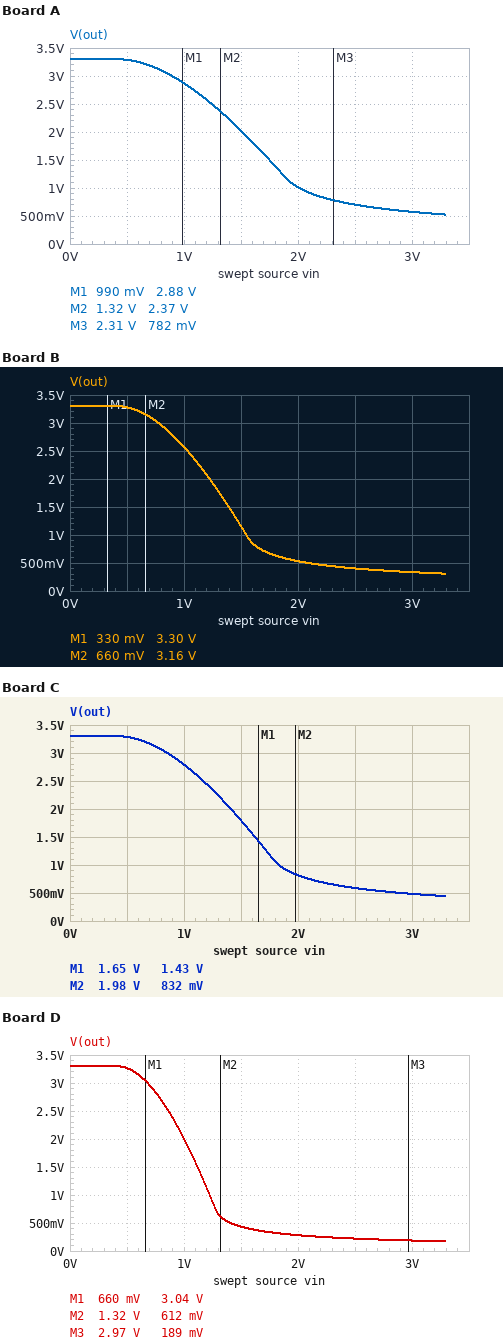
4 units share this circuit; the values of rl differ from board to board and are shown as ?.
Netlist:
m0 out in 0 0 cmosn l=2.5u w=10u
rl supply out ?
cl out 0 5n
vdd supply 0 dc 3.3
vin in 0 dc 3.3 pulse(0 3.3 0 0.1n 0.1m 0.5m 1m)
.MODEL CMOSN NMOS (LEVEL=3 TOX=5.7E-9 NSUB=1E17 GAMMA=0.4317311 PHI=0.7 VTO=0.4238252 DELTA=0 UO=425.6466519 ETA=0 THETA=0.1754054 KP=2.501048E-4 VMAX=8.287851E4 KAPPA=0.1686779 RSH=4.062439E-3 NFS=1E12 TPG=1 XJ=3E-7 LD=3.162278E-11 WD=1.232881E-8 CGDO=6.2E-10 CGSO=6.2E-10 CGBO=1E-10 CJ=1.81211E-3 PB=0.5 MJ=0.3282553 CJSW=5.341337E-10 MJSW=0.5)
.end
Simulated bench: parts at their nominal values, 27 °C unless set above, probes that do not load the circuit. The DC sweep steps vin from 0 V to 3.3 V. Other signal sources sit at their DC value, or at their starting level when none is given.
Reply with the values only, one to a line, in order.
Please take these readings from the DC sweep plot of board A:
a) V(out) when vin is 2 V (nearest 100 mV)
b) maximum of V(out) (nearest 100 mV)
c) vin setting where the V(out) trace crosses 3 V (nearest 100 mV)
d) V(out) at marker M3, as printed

1.0 V
3.3 V
900 mV
782 mV
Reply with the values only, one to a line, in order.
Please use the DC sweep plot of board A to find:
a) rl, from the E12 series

3.3 kΩ
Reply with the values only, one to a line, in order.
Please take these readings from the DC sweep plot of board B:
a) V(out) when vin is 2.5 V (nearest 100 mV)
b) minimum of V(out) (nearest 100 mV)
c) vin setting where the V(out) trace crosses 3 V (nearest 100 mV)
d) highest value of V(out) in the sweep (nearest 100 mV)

400 mV
300 mV
800 mV
3.3 V
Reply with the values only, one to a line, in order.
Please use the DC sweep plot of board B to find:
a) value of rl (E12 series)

5.6 kΩ
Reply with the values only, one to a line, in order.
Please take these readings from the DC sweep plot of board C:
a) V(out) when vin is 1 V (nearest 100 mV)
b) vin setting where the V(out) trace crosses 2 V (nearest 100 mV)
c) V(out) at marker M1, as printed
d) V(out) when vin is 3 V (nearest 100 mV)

2.8 V
1.4 V
1.43 V
500 mV
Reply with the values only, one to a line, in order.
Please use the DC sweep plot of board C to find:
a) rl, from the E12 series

3.9 kΩ
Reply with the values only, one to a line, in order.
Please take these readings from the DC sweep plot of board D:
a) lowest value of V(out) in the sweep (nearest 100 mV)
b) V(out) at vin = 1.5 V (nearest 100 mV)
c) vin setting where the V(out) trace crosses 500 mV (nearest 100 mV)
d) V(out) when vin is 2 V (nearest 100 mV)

200 mV
400 mV
1.4 V
300 mV
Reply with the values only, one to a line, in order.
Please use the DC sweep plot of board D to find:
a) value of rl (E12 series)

10 kΩ
